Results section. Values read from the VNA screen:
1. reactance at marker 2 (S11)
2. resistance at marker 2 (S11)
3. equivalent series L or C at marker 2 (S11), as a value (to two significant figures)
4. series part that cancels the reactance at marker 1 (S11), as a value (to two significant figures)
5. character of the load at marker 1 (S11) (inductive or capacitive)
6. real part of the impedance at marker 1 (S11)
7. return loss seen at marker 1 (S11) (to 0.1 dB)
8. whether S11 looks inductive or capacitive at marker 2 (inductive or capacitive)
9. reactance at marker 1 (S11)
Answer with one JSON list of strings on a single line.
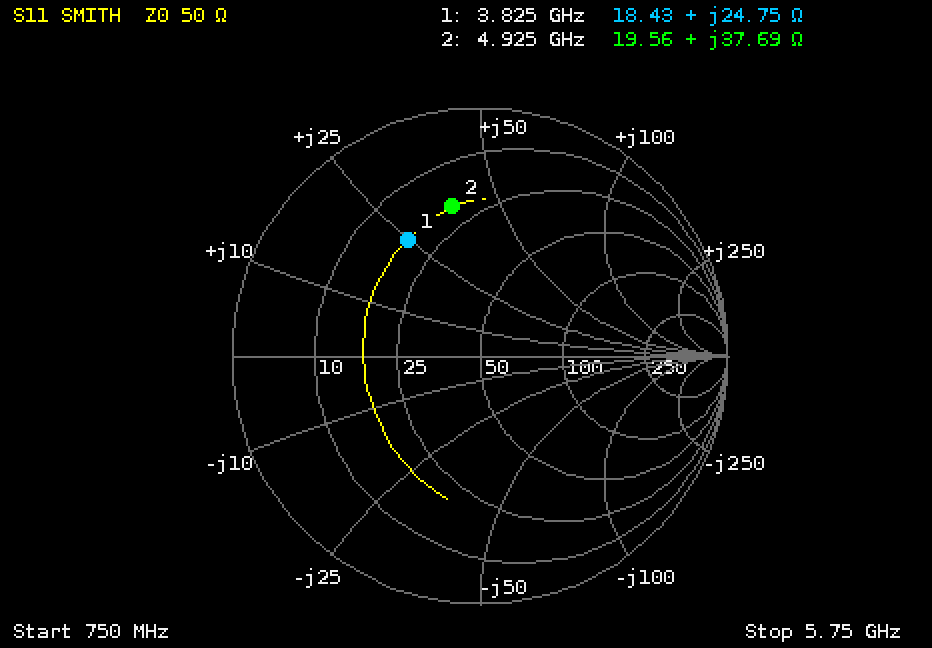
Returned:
["+37.69 Ω", "19.56 Ω", "1.2 nH", "1.7 pF", "inductive", "18.43 Ω", "5.2 dB", "inductive", "+24.75 Ω"]
